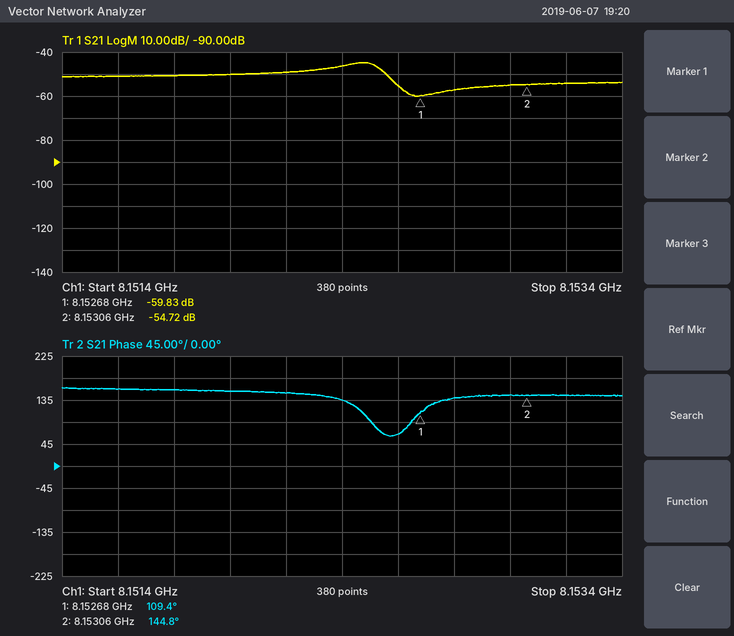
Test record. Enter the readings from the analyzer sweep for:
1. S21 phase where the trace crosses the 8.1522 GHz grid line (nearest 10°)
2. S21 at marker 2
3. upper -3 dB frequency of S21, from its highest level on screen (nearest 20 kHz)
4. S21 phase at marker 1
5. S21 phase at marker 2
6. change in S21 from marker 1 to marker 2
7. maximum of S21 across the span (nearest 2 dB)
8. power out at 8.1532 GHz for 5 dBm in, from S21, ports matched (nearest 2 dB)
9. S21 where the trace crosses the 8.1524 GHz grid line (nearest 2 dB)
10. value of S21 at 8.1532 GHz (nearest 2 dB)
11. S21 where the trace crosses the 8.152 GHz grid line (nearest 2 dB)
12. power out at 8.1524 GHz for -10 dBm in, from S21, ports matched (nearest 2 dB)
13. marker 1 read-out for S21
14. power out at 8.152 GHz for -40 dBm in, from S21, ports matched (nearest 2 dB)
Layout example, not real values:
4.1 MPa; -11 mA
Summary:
150°; -54.72 dB; 8.15254 GHz; 109.4°; 144.8°; 5.11 dB; -44 dB; -50 dBm; -46 dB; -54 dB; -50 dB; -56 dBm; -59.83 dB; -90 dBm
